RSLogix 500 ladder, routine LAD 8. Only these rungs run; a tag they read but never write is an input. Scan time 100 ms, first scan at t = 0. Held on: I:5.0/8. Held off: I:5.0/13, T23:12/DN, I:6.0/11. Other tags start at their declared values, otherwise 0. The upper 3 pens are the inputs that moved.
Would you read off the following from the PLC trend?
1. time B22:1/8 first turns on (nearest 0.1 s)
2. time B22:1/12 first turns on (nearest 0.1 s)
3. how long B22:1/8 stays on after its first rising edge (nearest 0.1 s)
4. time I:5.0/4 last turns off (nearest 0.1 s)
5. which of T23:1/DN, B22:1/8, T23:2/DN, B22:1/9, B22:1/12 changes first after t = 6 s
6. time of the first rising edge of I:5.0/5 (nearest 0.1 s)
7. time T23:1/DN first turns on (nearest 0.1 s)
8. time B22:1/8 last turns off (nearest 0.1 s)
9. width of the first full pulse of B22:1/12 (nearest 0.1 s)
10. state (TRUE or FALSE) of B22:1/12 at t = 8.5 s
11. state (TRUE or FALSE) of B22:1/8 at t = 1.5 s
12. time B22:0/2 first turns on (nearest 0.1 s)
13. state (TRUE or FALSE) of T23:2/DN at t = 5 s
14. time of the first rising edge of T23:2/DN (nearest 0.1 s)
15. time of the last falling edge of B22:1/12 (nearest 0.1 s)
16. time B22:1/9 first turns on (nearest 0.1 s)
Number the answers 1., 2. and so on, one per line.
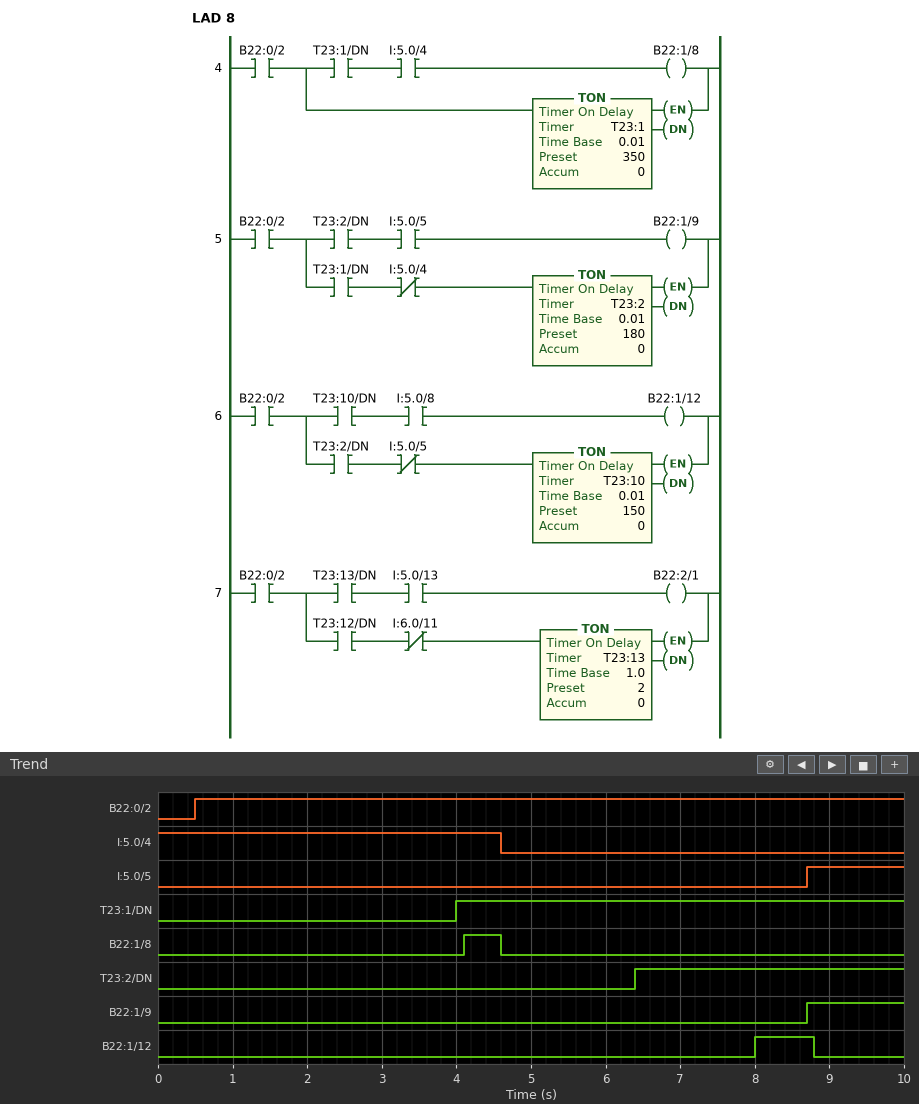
1. 4.1 s
2. 8.0 s
3. 0.5 s
4. 4.6 s
5. T23:2/DN
6. 8.7 s
7. 4.0 s
8. 4.6 s
9. 0.8 s
10. TRUE
11. FALSE
12. 0.5 s
13. FALSE
14. 6.4 s
15. 8.8 s
16. 8.7 s
